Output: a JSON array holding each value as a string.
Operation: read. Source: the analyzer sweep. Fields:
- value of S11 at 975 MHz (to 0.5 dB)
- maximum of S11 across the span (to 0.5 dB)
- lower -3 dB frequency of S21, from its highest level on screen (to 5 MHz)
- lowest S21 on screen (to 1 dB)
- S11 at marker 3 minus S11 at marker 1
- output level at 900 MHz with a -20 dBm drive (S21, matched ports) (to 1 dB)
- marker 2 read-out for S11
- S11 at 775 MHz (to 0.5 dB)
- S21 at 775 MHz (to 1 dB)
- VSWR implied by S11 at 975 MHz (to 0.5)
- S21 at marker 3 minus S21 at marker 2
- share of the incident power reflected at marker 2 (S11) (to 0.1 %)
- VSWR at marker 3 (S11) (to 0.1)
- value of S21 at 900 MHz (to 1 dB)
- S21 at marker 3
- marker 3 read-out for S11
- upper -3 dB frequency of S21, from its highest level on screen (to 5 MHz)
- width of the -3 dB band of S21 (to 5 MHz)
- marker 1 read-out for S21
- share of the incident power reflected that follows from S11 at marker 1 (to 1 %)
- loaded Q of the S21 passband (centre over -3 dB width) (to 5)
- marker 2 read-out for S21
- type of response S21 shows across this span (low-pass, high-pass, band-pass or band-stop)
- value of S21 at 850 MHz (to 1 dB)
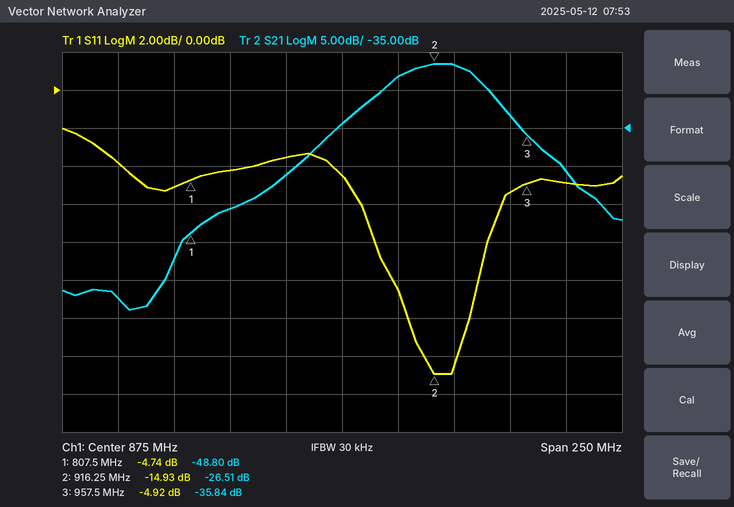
["-5.0 dB", "-2.0 dB", "895 MHz", "-59 dB", "-0.18 dB", "-48 dBm", "-14.93 dB", "-4.0 dB", "-57 dB", "3.5", "-9.33 dB", "3.2 %", "3.6", "-28 dB", "-35.84 dB", "-4.92 dB", "940 MHz", "45 MHz", "-48.80 dB", "34 %", "20", "-26.51 dB", "band-pass", "-41 dB"]
